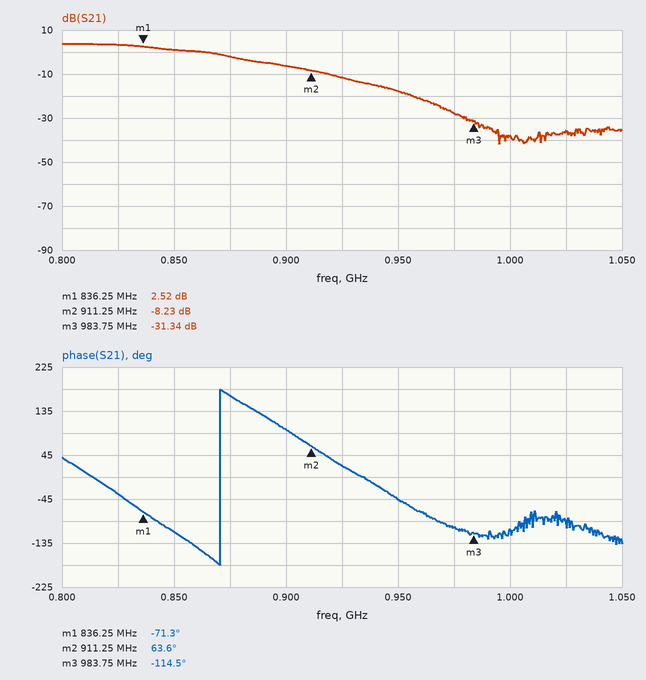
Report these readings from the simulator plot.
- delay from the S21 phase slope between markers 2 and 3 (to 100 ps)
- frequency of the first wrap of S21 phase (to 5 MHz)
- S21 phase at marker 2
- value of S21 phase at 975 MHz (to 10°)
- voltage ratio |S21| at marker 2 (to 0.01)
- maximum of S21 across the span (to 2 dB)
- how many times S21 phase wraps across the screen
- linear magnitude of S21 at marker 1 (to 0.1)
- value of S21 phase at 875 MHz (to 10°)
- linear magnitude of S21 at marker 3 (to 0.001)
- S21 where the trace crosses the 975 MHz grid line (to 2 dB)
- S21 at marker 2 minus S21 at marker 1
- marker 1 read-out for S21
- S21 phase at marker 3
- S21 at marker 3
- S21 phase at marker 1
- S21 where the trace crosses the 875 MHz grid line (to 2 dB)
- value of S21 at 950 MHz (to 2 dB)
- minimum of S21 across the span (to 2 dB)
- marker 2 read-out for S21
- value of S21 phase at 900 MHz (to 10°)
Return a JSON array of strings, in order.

["6.8 ns", "870 MHz", "63.6°", "-100°", "0.39", "4 dB", "1", "1.3", "170°", "0.027", "-28 dB", "-10.75 dB", "2.52 dB", "-114.5°", "-31.34 dB", "-71.3°", "-2 dB", "-18 dB", "-42 dB", "-8.23 dB", "100°"]
